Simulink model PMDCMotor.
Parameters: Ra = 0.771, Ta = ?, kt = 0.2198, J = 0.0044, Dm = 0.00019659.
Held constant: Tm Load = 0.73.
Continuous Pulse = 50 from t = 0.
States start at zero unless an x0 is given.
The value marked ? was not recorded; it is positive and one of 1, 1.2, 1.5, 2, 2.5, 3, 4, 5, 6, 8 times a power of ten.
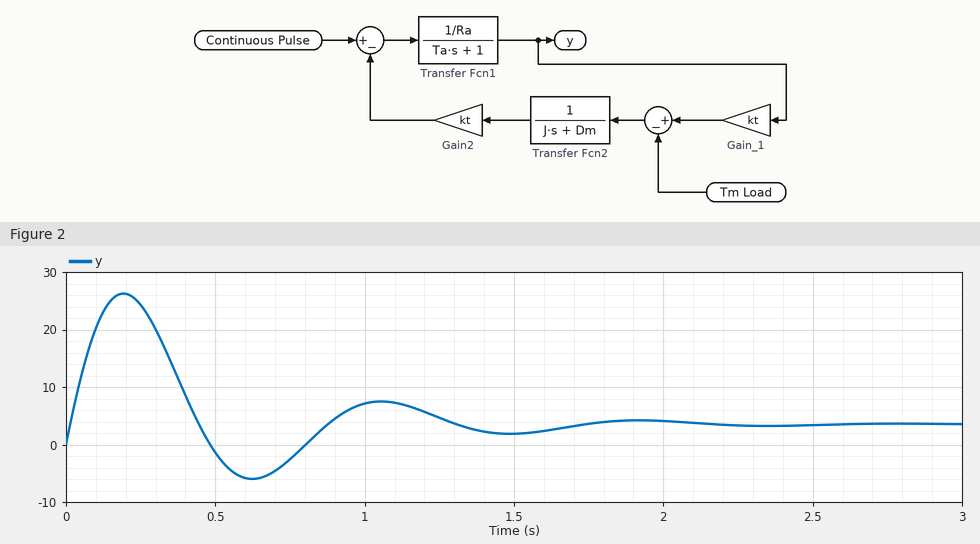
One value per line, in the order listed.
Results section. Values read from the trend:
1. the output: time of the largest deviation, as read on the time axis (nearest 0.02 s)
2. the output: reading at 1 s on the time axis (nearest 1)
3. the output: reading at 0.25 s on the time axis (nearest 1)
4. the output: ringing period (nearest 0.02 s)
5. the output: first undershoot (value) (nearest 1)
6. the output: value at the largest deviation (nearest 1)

0.20 s
7
24
0.86 s
-6
26
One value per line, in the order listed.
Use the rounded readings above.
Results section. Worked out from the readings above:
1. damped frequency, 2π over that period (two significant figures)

7.3 rad/s
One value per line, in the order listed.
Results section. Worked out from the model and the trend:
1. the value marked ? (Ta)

0.25
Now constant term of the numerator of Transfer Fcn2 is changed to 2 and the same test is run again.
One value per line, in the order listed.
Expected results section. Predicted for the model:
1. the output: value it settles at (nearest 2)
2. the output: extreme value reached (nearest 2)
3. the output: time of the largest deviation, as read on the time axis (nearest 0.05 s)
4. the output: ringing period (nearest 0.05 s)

4
22
0.15 s
0.60 s
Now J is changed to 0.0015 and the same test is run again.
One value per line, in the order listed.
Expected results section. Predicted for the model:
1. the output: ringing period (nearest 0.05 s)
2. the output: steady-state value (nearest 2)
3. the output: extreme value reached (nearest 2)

0.50 s
4
18
